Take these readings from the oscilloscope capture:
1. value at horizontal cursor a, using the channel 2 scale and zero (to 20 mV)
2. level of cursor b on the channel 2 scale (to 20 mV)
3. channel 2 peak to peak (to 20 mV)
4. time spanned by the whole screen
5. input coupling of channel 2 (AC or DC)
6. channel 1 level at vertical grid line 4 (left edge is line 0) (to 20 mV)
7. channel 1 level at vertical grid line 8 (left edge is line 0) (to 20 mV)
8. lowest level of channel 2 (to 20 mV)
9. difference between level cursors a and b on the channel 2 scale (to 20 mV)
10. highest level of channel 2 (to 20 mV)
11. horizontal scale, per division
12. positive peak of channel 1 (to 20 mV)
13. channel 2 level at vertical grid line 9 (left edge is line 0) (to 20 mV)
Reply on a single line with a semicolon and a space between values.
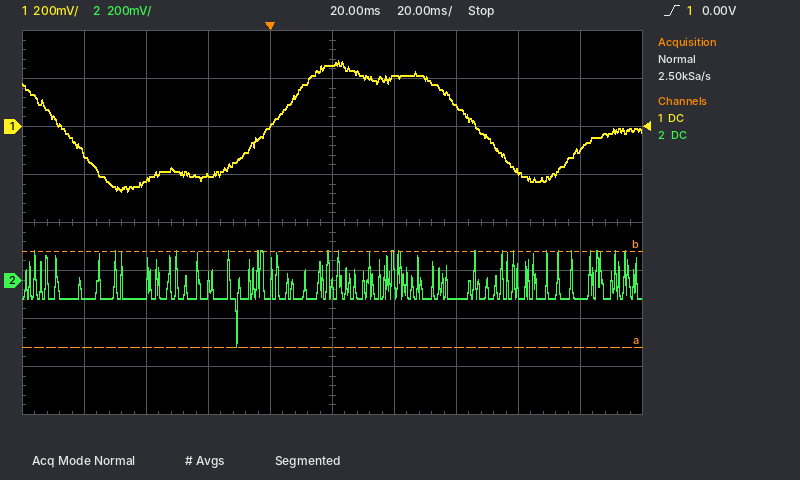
-280 mV; 120 mV; 400 mV; 200 ms; DC; 0 mV; -180 mV; -280 mV; 400 mV; 120 mV; 20 ms; 280 mV; -80 mV
